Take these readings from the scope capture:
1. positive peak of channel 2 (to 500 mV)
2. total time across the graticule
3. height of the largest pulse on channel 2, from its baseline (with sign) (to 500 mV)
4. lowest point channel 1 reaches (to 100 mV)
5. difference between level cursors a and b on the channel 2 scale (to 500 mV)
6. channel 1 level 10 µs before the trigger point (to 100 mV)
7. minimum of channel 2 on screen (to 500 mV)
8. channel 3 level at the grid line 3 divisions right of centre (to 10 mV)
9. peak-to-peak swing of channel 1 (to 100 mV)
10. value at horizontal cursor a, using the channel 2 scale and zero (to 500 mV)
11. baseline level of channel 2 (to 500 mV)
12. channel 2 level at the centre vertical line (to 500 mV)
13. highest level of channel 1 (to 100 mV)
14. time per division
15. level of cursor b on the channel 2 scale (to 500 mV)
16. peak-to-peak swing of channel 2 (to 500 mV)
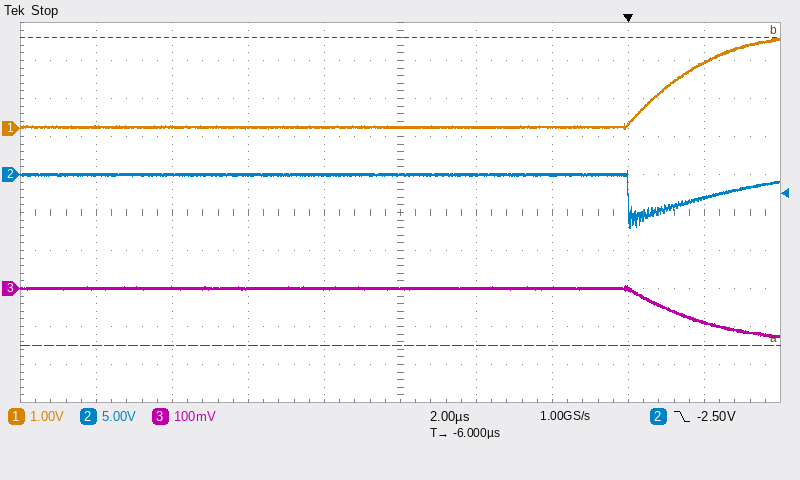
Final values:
500 mV
20 µs
-7.0 V
0.0 V
40.5 V
0.0 V
-7.0 V
0 mV
2.4 V
-22.5 V
0.0 V
0.0 V
2.4 V
2 µs
18.0 V
7.5 V
